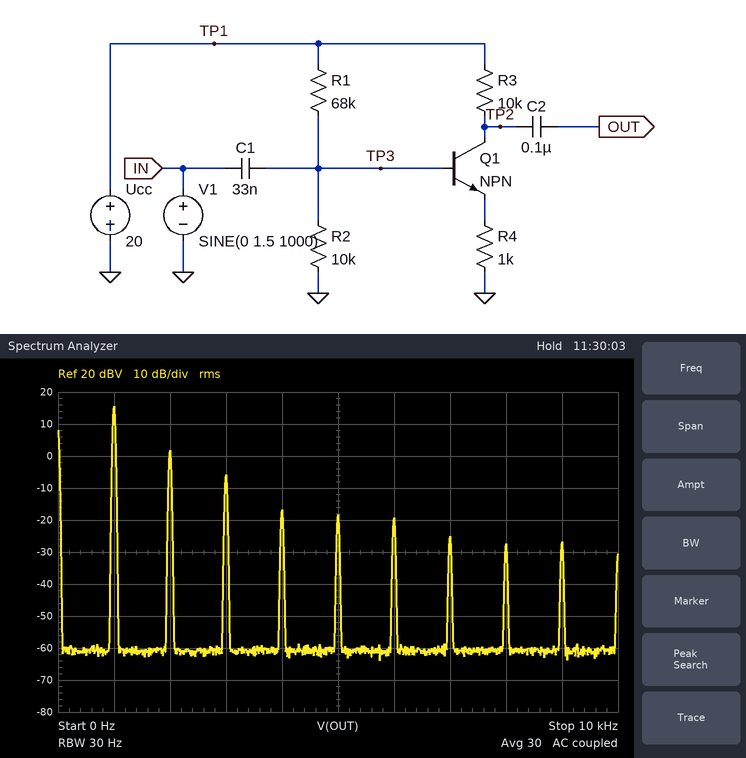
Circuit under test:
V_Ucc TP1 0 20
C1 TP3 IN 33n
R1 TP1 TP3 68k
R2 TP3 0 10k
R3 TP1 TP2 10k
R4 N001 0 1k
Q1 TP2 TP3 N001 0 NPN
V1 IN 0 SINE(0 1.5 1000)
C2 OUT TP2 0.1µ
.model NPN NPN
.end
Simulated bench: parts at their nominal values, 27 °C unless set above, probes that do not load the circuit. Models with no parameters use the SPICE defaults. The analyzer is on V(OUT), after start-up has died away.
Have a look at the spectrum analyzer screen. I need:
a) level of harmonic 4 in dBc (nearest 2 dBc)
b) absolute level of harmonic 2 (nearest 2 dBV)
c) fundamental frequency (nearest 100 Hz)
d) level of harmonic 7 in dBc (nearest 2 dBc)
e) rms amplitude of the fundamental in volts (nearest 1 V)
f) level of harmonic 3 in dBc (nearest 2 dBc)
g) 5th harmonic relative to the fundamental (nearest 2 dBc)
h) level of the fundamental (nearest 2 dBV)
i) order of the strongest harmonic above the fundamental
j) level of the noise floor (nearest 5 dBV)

-32 dBc
2 dBV
1.0 kHz
-40 dBc
6 V
-22 dBc
-34 dBc
16 dBV
2
-60 dBV
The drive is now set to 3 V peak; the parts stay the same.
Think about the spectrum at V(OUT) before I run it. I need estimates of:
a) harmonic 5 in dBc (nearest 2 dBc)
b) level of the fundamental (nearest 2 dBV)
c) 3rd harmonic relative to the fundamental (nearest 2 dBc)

-22 dBc
18 dBV
-12 dBc
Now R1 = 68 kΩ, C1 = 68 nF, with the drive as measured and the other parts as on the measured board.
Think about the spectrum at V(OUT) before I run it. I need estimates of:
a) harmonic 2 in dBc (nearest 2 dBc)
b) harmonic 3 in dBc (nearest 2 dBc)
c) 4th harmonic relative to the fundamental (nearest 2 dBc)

-18 dBc
-18 dBc
-30 dBc
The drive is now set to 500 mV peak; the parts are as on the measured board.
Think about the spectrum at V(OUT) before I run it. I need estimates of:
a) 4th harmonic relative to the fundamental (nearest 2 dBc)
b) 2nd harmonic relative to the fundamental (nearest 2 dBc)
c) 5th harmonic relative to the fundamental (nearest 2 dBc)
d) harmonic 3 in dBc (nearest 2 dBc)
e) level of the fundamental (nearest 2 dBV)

-30 dBc
-18 dBc
-38 dBc
-24 dBc
8 dBV
